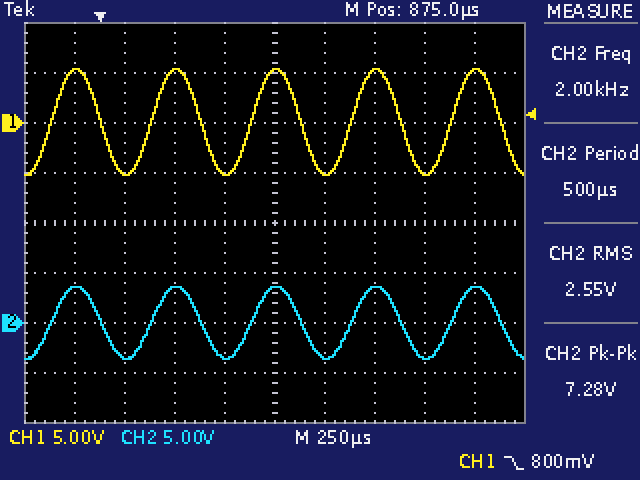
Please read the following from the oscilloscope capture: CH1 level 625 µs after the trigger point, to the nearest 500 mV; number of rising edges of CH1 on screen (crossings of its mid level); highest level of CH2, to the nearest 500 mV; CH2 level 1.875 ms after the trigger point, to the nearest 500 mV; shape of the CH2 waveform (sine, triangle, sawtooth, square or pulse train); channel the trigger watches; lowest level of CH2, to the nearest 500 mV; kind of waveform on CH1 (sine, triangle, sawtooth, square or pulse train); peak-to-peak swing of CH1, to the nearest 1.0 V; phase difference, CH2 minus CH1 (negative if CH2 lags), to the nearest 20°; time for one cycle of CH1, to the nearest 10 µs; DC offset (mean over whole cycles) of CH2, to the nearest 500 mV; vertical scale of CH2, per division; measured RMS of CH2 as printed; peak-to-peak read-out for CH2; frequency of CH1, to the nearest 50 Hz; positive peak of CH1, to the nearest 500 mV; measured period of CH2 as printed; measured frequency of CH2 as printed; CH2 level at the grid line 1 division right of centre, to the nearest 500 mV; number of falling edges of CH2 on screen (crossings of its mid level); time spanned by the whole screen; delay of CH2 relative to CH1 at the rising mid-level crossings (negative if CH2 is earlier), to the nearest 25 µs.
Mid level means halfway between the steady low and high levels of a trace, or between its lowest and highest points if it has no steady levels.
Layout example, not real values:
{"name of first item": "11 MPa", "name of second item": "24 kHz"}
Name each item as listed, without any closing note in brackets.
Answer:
{"CH1 level 625 µs after the trigger point, to the nearest 500 mV": "-5.0 V", "number of rising edges of CH1 on screen": "5", "highest level of CH2, to the nearest 500 mV": "3.5 V", "CH2 level 1.875 ms after the trigger point, to the nearest 500 mV": "3.5 V", "shape of the CH2 waveform": "sine", "channel the trigger watches": "CH1", "lowest level of CH2, to the nearest 500 mV": "-3.5 V", "kind of waveform on CH1": "sine", "peak-to-peak swing of CH1, to the nearest 1.0 V": "11.0 V", "phase difference, CH2 minus CH1 (negative if CH2 lags), to the nearest 20°": "0°", "time for one cycle of CH1, to the nearest 10 µs": "500 µs", "DC offset (mean over whole cycles) of CH2, to the nearest 500 mV": "0.0 V", "vertical scale of CH2, per division": "5 V", "measured RMS of CH2 as printed": "2.55 V", "peak-to-peak read-out for CH2": "7.28 V", "frequency of CH1, to the nearest 50 Hz": "2.00 kHz", "positive peak of CH1, to the nearest 500 mV": "5.5 V", "measured period of CH2 as printed": "500 µs", "measured frequency of CH2 as printed": "2.00 kHz", "CH2 level at the grid line 1 division right of centre, to the nearest 500 mV": "-3.5 V", "number of falling edges of CH2 on screen": "5", "time spanned by the whole screen": "2.5 ms", "delay of CH2 relative to CH1 at the rising mid-level crossings (negative if CH2 is earlier), to the nearest 25 µs": "0 µs"}
